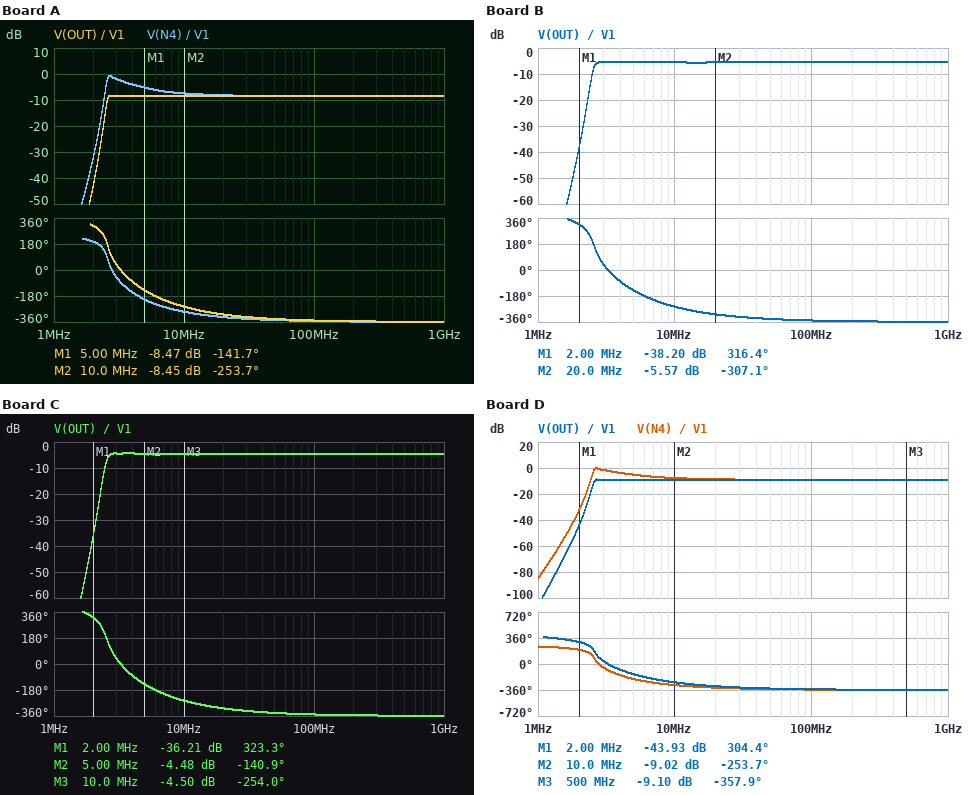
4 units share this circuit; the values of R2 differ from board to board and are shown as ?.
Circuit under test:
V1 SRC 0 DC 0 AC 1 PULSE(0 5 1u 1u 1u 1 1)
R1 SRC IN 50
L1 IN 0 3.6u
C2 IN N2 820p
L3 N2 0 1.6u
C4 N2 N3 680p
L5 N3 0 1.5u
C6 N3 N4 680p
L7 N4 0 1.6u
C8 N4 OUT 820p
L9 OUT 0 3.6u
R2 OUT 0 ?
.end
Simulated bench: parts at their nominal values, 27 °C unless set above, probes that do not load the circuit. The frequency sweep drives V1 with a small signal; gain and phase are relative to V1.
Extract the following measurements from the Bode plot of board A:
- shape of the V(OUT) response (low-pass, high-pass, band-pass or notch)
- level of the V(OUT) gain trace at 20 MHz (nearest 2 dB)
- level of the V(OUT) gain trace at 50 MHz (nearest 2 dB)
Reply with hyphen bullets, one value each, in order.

- high-pass
- -8 dB
- -8 dB
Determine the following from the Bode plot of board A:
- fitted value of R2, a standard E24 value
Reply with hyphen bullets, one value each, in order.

- 30 Ω
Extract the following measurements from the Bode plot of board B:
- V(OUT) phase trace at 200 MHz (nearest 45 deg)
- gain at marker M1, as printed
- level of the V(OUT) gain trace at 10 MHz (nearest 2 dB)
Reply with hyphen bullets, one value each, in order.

- -360 deg
- -38.20 dB
- -6 dB
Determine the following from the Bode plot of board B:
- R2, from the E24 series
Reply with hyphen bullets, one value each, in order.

- 56 Ω
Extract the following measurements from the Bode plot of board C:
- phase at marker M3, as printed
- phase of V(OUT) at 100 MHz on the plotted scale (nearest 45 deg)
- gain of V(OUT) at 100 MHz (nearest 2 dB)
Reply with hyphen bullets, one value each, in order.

- -254.0 deg
- -360 deg
- -4 dB
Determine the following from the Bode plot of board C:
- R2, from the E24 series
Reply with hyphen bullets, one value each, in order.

- 75 Ω
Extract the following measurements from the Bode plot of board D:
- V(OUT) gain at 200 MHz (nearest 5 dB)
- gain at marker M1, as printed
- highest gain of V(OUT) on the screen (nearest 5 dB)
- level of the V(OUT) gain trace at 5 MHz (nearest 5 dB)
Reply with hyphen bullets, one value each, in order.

- -10 dB
- -43.93 dB
- -10 dB
- -10 dB
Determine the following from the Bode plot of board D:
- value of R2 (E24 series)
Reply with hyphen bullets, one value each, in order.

- 27 Ω
